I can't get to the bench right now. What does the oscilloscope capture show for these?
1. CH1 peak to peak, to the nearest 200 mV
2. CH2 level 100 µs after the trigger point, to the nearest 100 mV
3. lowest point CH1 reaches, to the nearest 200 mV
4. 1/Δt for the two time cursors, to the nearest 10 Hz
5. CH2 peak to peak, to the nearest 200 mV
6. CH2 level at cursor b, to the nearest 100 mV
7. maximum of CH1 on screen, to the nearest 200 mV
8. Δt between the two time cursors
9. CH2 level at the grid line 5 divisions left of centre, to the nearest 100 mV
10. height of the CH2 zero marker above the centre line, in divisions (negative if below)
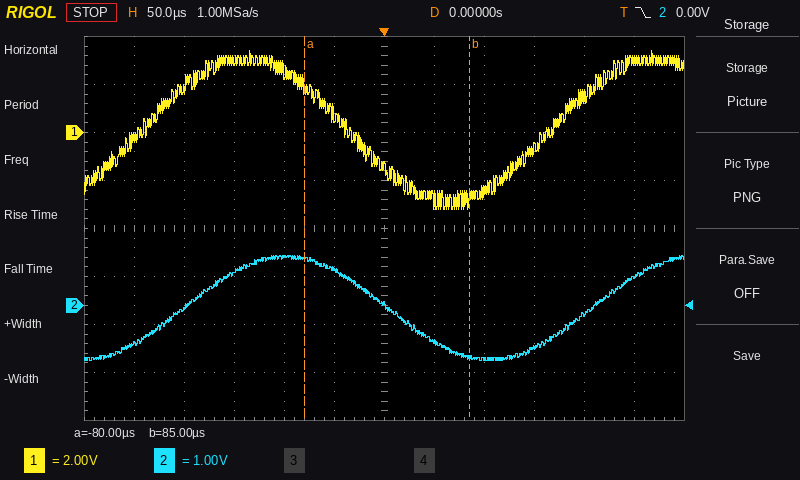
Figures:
6.6 V
-1.1 V
-3.2 V
6.06 kHz
2.2 V
-1.1 V
3.4 V
165 µs
-800 mV
-1.6 div
